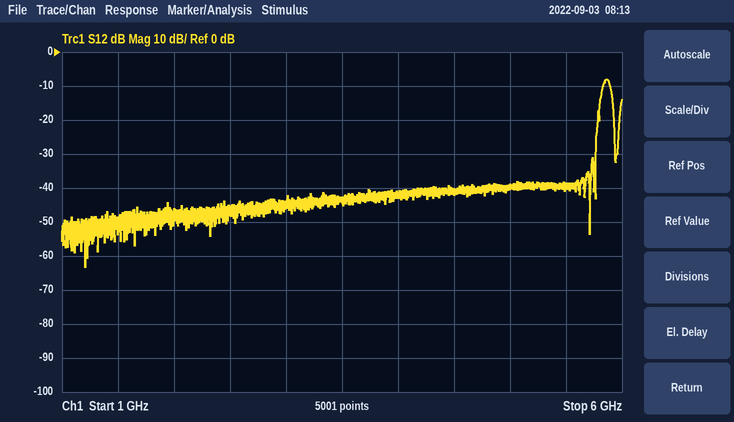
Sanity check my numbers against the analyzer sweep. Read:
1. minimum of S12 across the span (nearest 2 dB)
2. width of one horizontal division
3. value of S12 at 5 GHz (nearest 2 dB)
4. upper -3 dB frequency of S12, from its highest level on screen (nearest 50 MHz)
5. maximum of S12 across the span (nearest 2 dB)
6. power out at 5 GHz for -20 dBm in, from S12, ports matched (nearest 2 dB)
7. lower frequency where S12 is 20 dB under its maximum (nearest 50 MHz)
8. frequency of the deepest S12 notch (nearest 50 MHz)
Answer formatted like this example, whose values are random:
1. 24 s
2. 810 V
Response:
1. -64 dB
2. 500 MHz
3. -40 dB
4. 5.90 GHz
5. -8 dB
6. -60 dBm
7. 5.75 GHz
8. 1.20 GHz
